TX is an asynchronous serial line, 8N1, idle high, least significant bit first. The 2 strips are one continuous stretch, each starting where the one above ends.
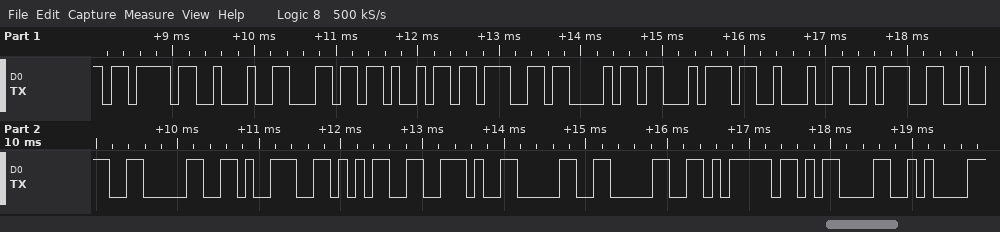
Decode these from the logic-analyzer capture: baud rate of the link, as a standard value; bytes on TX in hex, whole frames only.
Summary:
9600 baud
0x7B 0x22 0x6C 0x69 0x67 0x68 0x74 0x22 0x3A 0x32 0x30 0x39 0x35 0x2E 0x30 0x30 0x7D 0x0D 0x0A
